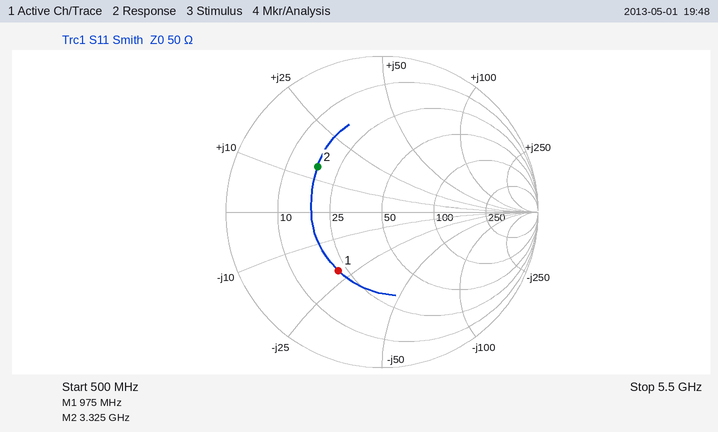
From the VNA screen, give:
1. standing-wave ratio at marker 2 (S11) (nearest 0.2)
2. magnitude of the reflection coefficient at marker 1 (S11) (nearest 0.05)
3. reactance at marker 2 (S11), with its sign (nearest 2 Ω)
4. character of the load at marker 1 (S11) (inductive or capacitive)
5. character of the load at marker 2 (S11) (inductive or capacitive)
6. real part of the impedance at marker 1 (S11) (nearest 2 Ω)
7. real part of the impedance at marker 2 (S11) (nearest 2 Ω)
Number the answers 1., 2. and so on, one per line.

1. 3.0
2. 0.45
3. +14 Ω
4. capacitive
5. inductive
6. 22 Ω
7. 18 Ω
